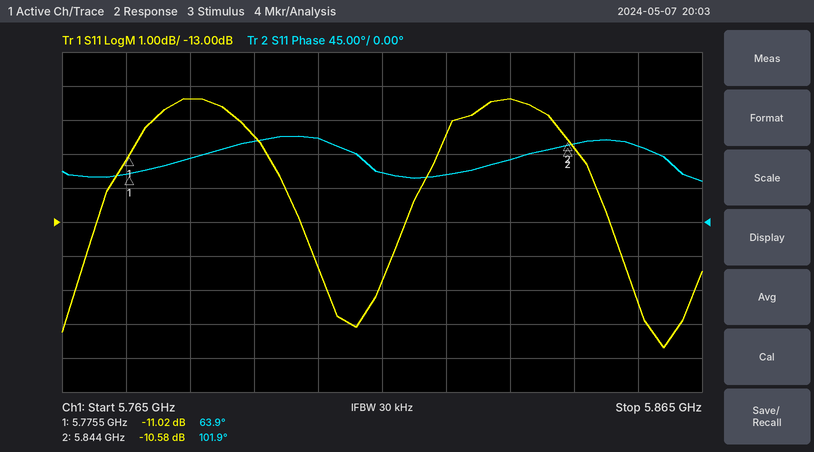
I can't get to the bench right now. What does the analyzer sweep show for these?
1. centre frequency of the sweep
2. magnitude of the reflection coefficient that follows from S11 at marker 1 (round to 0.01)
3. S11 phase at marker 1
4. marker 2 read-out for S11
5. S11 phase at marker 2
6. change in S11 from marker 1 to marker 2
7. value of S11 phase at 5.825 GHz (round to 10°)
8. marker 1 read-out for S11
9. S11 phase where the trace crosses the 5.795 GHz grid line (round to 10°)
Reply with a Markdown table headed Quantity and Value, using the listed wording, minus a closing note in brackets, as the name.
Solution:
| Quantity | Value |
|---|---|
| centre frequency of the sweep | 5.815 GHz |
| magnitude of the reflection coefficient that follows from S11 at marker 1 | 0.28 |
| S11 phase at marker 1 | 63.9° |
| marker 2 read-out for S11 | -10.58 dB |
| S11 phase at marker 2 | 101.9° |
| change in S11 from marker 1 to marker 2 | 0.44 dB |
| value of S11 phase at 5.825 GHz | 60° |
| marker 1 read-out for S11 | -11.02 dB |
| S11 phase where the trace crosses the 5.795 GHz grid line | 110° |
